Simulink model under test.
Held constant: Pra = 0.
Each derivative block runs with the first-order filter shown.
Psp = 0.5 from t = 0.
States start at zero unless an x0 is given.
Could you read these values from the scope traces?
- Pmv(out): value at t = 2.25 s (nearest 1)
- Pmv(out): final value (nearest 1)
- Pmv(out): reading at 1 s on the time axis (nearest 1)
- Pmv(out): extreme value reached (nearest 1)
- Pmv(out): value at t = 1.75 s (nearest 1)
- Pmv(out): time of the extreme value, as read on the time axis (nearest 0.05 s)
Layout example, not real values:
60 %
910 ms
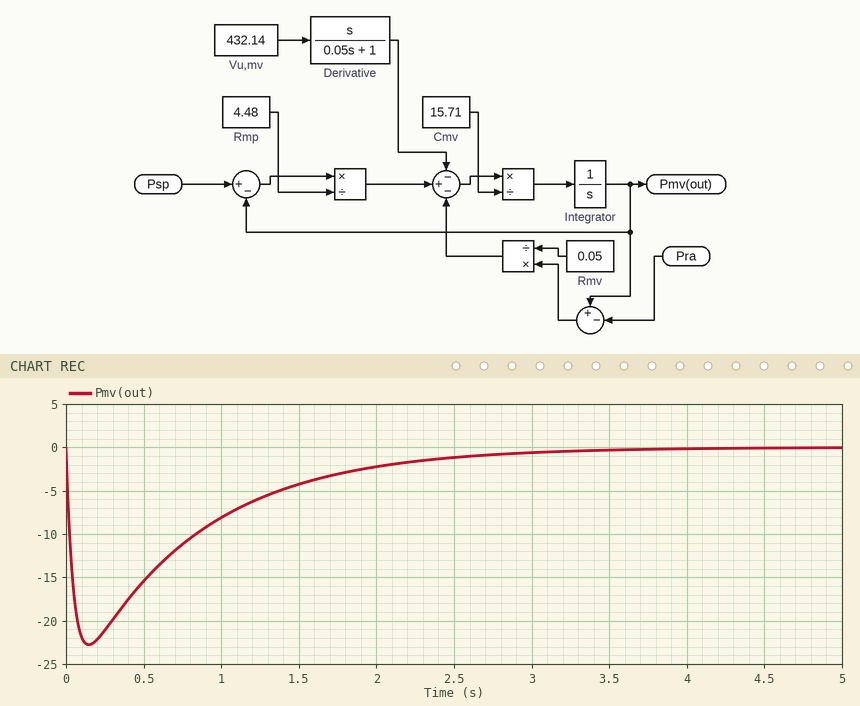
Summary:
-2
0
-8
-23
-3
0.15 s
